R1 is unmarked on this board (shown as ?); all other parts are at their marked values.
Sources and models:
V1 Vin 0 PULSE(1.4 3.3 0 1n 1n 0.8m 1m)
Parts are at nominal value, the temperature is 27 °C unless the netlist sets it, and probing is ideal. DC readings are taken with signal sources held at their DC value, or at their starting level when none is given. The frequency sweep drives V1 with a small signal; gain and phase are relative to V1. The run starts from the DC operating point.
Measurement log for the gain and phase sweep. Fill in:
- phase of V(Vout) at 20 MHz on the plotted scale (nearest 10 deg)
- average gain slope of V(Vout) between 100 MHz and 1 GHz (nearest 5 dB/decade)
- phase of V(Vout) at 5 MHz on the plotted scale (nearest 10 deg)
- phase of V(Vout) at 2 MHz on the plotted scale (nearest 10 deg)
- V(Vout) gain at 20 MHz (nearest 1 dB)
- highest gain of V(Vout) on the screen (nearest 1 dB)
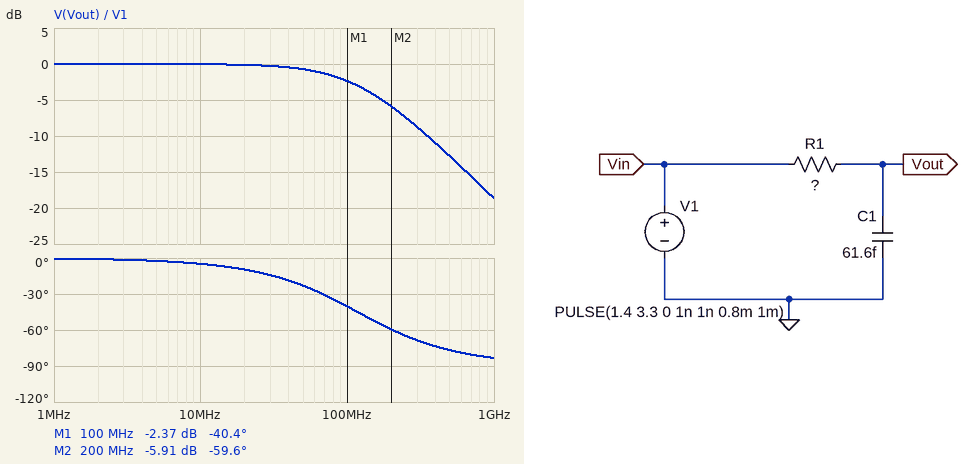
-10 deg
-15 dB/decade
0 deg
0 deg
0 dB
0 dB
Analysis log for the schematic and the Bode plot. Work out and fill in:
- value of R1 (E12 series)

22 kΩ
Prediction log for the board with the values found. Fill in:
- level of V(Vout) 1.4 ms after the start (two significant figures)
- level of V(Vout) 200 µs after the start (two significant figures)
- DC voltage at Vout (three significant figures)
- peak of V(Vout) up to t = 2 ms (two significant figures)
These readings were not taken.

3.3 V
3.3 V
1.40 V
3.3 V
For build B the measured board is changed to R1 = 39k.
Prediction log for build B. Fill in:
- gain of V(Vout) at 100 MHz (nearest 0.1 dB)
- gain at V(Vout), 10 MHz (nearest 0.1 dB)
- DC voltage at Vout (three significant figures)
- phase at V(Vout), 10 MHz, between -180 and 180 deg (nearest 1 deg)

-5.2 dB
-0.1 dB
1.40 V
-9 deg
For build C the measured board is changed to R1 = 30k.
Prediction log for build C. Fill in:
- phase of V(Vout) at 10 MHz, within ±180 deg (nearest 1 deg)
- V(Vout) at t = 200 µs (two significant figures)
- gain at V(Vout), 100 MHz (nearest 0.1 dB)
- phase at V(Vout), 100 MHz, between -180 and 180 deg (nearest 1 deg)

-7 deg
3.3 V
-3.7 dB
-49 deg
